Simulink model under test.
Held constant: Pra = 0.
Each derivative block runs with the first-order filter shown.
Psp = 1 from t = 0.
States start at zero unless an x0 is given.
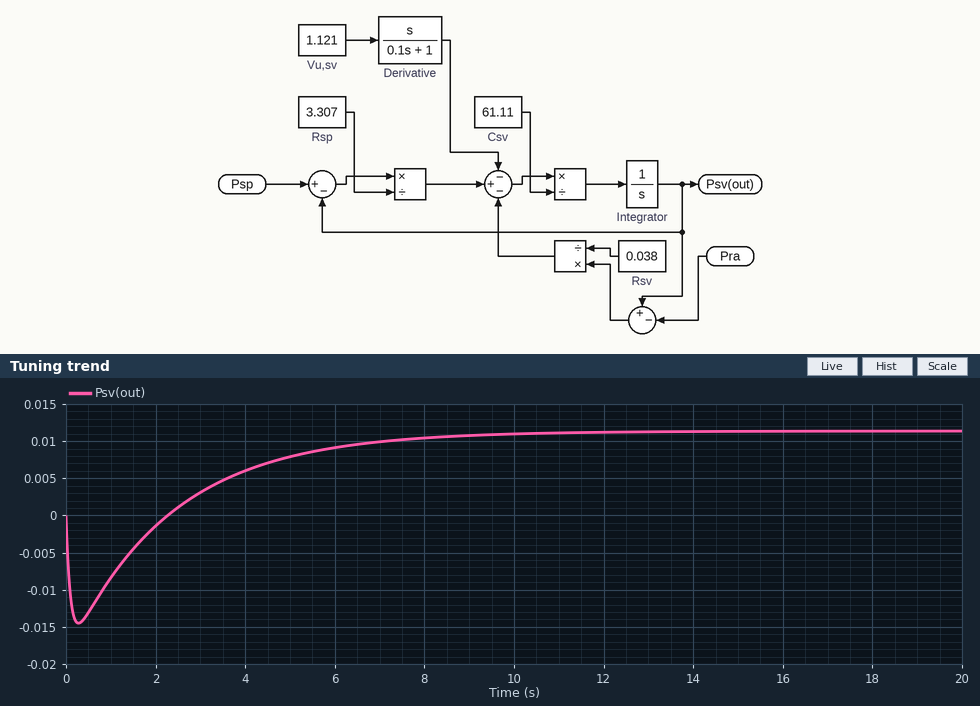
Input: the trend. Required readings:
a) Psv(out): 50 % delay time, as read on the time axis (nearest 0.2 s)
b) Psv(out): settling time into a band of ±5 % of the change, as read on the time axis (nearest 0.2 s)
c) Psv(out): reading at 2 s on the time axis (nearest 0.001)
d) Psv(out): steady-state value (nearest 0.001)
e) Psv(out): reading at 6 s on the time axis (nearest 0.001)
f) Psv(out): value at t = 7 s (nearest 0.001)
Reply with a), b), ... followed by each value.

a) 3.8 s
b) 9.2 s
c) -0.001
d) 0.011
e) 0.009
f) 0.010
